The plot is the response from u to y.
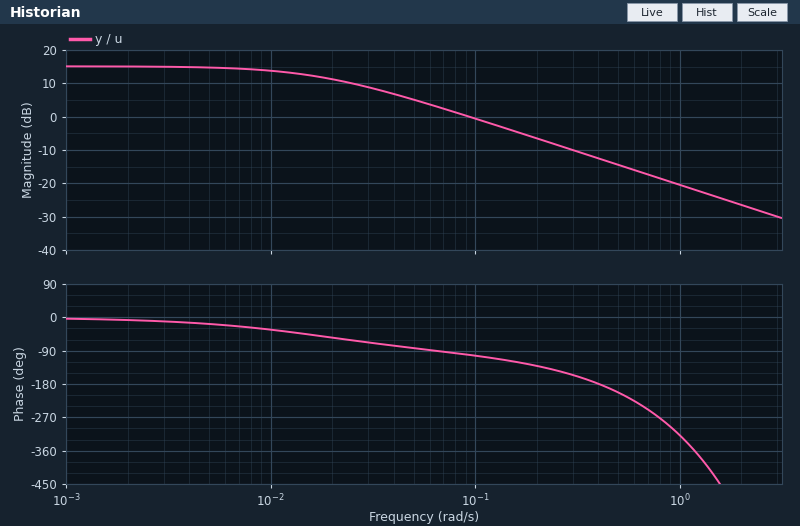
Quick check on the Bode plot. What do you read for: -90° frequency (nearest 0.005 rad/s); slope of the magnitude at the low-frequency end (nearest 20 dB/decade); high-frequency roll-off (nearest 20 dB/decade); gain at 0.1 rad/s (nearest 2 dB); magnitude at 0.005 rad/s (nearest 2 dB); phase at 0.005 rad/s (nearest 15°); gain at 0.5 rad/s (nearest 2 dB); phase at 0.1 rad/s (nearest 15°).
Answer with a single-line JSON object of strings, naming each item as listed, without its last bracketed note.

{"-90° frequency": "0.065 rad/s", "slope of the magnitude at the low-frequency end": "0 dB/decade", "high-frequency roll-off": "-20 dB/decade", "gain at 0.1 rad/s": "0 dB", "magnitude at 0.005 rad/s": "14 dB", "phase at 0.005 rad/s": "-15°", "gain at 0.5 rad/s": "-14 dB", "phase at 0.1 rad/s": "-105°"}
